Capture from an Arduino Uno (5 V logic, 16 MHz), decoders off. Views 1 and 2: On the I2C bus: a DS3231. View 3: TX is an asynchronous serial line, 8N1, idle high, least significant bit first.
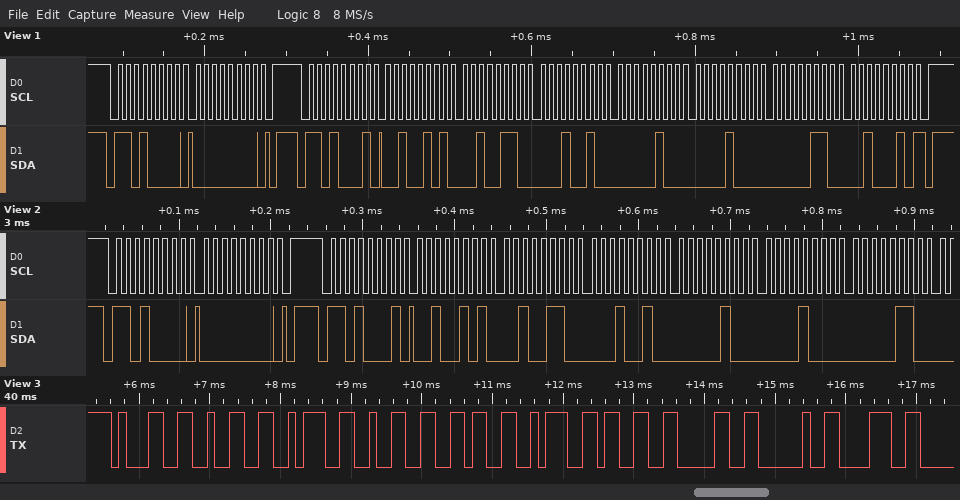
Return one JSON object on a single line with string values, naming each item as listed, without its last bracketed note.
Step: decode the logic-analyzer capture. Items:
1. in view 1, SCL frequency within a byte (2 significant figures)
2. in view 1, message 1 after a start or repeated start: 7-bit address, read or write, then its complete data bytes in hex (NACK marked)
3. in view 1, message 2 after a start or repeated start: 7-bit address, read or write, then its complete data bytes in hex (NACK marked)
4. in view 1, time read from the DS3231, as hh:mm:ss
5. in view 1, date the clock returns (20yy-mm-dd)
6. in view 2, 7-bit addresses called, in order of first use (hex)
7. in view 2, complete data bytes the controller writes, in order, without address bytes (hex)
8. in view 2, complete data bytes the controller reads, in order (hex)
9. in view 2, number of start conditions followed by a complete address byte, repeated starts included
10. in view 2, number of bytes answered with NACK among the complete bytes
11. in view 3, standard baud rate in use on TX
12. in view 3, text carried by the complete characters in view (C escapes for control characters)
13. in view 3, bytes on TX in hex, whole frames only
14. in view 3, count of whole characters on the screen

{"in view 1, SCL frequency within a byte": "100 kHz", "in view 1, message 1 after a start or repeated start: 7-bit address, read or write, then its complete data bytes in hex": "0x68 write: 00", "in view 1, message 2 after a start or repeated start: 7-bit address, read or write, then its complete data bytes in hex": "0x68 read: 25 26 12 04 08 06 22 NACK", "in view 1, time read from the DS3231, as hh:mm:ss": "12:26:25", "in view 1, date the clock returns": "2022-06-08", "in view 2, 7-bit addresses called, in order of first use": "0x68", "in view 2, complete data bytes the controller writes, in order, without address bytes": "00", "in view 2, complete data bytes the controller reads, in order": "25 26 12 04 08 06", "in view 2, number of start conditions followed by a complete address byte, repeated starts included": "2", "in view 2, number of bytes answered with NACK among the complete bytes": "0", "in view 3, standard baud rate in use on TX": "9600 baud", "in view 3, text carried by the complete characters in view": "\"12:26:30 8\"", "in view 3, bytes on TX in hex, whole frames only": "31 32 3A 32 36 3A 33 30 20 38", "in view 3, count of whole characters on the screen": "10"}
